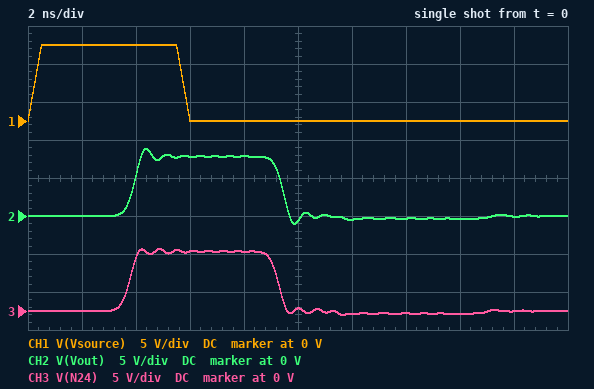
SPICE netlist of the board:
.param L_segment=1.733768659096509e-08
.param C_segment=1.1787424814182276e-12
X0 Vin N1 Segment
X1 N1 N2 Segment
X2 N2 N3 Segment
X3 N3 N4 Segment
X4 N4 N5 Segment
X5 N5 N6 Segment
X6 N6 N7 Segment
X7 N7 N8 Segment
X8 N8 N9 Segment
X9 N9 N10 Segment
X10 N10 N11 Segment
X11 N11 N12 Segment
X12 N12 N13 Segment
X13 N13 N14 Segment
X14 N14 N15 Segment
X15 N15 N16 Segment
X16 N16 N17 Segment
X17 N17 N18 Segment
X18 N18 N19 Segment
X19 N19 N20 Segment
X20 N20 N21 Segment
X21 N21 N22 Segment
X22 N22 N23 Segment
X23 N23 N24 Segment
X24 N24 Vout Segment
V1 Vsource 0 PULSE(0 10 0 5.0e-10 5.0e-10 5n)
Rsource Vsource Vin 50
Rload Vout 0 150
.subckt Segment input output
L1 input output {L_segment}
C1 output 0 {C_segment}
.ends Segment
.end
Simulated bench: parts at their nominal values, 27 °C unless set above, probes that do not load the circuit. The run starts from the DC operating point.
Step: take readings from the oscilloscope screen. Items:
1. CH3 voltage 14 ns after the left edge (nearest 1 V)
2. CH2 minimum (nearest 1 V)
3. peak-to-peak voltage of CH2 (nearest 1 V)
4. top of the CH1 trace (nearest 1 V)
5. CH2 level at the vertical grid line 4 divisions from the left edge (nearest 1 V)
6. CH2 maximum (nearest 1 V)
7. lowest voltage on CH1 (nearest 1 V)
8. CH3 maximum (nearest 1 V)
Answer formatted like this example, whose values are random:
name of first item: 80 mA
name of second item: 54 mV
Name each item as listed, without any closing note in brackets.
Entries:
CH3 voltage 14 ns after the left edge: 0 V
CH2 minimum: -1 V
peak-to-peak voltage of CH2: 10 V
top of the CH1 trace: 10 V
CH2 level at the vertical grid line 4 divisions from the left edge: 8 V
CH2 maximum: 9 V
lowest voltage on CH1: 0 V
CH3 maximum: 8 V
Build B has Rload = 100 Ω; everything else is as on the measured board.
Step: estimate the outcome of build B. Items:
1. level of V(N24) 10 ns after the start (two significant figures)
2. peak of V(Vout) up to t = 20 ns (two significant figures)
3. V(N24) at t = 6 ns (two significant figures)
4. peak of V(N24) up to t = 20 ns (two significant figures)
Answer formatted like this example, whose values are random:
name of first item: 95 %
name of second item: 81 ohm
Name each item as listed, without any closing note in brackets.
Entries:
level of V(N24) 10 ns after the start: 530 mV
peak of V(Vout) up to t = 20 ns: 7.2 V
V(N24) at t = 6 ns: 6.4 V
peak of V(N24) up to t = 20 ns: 7.1 V
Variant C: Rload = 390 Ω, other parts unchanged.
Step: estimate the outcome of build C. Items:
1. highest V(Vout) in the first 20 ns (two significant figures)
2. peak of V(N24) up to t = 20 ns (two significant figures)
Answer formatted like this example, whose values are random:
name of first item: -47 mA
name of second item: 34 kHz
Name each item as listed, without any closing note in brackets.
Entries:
highest V(Vout) in the first 20 ns: 12 V
peak of V(N24) up to t = 20 ns: 11 V
